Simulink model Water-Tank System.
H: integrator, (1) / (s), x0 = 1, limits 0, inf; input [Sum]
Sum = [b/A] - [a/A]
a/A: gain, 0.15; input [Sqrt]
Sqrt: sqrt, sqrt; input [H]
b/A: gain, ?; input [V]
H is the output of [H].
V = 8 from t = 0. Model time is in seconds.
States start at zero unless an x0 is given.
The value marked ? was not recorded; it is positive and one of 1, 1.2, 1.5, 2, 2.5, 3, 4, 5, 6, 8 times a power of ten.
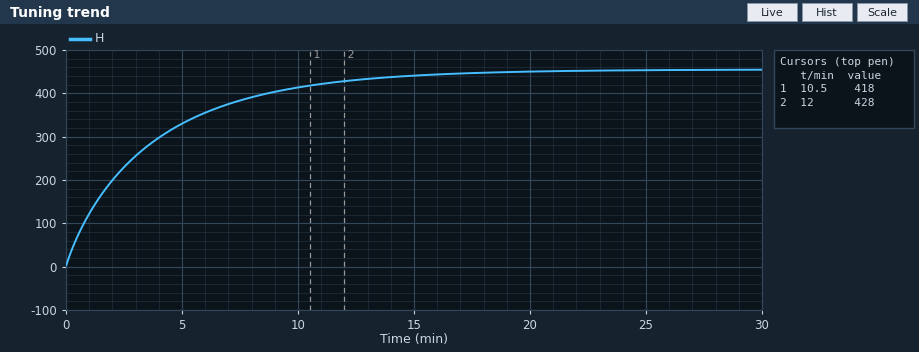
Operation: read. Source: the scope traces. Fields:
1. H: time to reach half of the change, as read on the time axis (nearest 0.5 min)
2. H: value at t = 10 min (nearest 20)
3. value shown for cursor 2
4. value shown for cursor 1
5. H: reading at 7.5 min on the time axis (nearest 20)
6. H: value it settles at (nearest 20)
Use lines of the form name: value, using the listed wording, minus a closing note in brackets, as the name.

H: time to reach half of the change, as read on the time axis: 2.5 min
H: value at t = 10 min: 420
value shown for cursor 2: 428
value shown for cursor 1: 418
H: reading at 7.5 min on the time axis: 380
H: value it settles at: 460
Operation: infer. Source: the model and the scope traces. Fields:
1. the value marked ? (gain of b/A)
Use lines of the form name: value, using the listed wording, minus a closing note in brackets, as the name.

the value marked ?: 0.4
